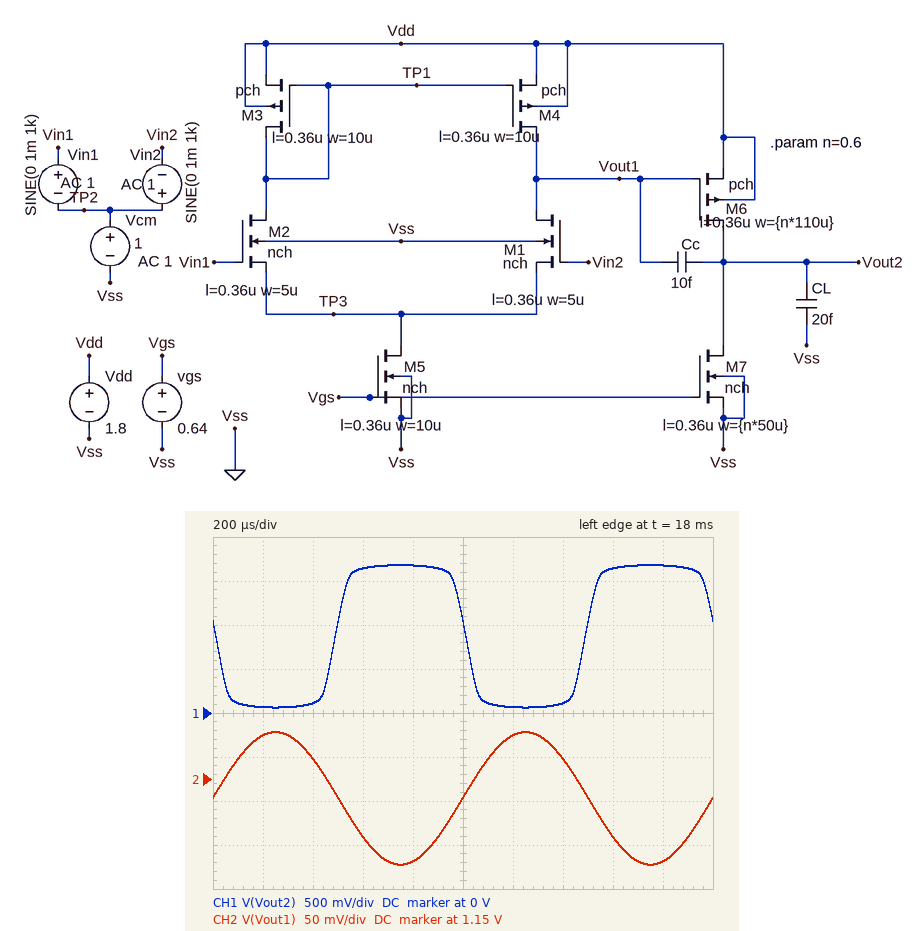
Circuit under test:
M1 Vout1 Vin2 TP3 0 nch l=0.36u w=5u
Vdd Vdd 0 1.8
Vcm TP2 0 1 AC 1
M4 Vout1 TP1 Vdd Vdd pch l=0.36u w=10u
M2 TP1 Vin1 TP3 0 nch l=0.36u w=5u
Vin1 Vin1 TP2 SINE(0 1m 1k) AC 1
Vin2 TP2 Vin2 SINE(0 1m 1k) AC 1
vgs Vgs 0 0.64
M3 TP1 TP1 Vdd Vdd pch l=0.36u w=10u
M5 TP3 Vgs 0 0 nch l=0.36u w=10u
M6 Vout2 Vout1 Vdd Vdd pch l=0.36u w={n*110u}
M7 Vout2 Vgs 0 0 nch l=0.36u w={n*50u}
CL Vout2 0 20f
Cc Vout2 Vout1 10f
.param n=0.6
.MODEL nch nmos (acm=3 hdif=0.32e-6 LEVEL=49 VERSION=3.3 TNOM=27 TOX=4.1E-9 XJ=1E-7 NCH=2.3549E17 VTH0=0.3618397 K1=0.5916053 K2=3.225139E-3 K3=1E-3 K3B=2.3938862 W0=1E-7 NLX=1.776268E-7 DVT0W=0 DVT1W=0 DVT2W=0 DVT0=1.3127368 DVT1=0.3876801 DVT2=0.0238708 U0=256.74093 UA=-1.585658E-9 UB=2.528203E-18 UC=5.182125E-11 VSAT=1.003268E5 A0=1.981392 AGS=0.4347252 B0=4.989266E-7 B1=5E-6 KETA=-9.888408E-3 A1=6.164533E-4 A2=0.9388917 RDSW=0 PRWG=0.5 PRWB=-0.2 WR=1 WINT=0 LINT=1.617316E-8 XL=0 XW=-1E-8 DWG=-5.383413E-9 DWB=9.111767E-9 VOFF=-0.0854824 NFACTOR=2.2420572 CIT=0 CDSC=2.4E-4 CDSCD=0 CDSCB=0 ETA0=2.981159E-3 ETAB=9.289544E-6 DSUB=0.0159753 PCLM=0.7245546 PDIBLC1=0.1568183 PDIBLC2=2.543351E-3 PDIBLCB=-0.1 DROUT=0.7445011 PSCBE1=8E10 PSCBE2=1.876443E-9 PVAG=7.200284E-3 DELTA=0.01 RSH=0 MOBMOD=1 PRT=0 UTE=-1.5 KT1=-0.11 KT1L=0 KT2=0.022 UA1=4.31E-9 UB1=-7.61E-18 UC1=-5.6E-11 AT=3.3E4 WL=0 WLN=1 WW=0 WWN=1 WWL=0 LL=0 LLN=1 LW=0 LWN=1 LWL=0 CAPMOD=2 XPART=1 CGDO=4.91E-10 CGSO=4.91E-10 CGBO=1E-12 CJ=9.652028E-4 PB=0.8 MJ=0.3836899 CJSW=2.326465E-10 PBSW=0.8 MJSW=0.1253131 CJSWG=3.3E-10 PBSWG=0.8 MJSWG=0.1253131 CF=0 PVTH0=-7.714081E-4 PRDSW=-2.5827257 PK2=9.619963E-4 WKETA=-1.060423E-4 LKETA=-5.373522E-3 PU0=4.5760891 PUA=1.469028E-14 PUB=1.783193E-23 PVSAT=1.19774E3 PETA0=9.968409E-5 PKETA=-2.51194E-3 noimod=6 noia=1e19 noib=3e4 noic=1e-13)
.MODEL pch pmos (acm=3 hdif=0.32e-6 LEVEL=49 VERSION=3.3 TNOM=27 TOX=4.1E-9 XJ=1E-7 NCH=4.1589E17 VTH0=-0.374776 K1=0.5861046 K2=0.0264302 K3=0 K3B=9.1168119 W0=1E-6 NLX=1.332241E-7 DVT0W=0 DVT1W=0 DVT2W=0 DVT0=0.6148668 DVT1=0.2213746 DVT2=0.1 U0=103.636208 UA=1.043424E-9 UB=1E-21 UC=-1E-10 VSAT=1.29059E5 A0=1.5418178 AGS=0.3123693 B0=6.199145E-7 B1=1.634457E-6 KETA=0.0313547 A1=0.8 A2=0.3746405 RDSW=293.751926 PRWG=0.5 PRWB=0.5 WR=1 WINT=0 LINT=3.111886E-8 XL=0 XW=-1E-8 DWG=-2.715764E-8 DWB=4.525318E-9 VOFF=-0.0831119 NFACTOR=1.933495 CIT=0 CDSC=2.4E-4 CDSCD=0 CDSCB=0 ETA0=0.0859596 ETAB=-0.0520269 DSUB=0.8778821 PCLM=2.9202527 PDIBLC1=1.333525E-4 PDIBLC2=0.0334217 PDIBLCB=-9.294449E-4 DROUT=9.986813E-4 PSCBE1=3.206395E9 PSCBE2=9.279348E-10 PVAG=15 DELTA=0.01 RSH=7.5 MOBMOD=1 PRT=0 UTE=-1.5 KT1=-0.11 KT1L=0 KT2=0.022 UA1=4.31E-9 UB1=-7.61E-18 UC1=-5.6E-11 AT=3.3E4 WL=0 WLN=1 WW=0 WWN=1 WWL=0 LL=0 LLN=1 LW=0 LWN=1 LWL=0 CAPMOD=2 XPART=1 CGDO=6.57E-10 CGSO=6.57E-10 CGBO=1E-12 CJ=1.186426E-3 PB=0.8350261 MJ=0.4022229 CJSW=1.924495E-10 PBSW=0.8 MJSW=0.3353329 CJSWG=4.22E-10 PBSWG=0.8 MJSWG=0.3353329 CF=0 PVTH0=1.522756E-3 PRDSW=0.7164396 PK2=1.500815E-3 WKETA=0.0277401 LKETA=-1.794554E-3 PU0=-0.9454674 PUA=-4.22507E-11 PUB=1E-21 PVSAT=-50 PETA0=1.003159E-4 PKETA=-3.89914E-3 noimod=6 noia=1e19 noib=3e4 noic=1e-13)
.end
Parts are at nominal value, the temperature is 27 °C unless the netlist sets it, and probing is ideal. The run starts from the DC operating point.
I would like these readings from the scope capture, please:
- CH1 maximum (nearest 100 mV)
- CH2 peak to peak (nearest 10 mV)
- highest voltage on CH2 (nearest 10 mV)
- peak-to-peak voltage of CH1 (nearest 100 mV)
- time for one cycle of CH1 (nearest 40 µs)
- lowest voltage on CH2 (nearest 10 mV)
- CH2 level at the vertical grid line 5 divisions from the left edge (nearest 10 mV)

1.7 V
150 mV
1.20 V
1.6 V
1.00 ms
1.05 V
1.13 V
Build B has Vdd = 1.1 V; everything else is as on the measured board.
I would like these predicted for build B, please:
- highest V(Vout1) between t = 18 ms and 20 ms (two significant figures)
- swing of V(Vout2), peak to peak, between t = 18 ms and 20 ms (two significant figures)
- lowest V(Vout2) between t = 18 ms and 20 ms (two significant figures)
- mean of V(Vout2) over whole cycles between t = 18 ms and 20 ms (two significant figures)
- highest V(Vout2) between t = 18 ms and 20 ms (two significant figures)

440 mV
500 mV
330 mV
610 mV
830 mV
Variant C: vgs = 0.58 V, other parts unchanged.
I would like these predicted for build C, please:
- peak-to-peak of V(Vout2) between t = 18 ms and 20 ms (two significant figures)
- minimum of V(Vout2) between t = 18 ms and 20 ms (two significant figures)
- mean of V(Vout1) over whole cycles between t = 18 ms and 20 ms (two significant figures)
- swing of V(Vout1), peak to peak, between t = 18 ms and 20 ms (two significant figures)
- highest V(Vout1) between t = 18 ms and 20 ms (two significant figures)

1.7 V
29 mV
1.2 V
160 mV
1.3 V
